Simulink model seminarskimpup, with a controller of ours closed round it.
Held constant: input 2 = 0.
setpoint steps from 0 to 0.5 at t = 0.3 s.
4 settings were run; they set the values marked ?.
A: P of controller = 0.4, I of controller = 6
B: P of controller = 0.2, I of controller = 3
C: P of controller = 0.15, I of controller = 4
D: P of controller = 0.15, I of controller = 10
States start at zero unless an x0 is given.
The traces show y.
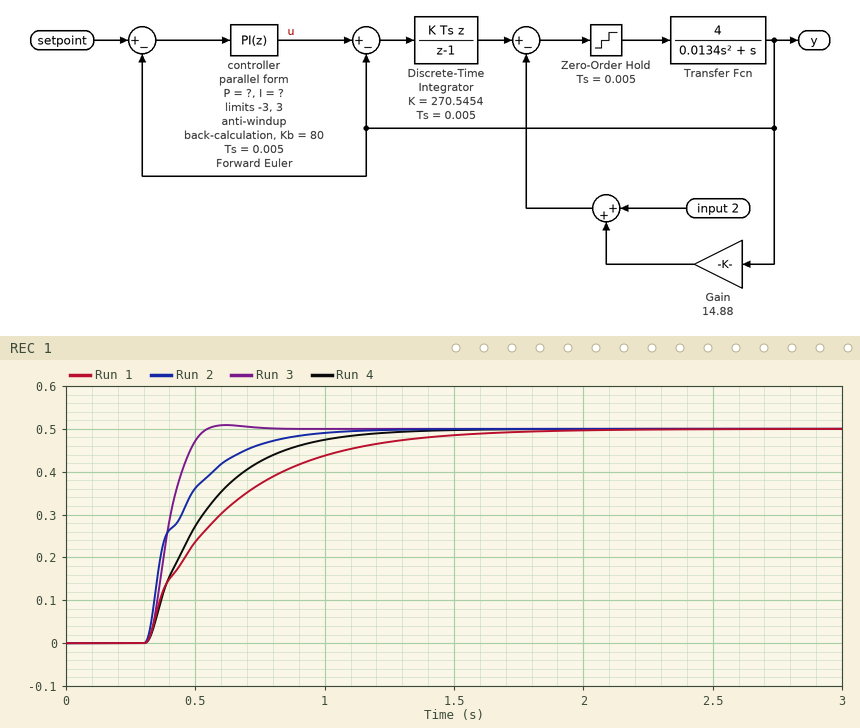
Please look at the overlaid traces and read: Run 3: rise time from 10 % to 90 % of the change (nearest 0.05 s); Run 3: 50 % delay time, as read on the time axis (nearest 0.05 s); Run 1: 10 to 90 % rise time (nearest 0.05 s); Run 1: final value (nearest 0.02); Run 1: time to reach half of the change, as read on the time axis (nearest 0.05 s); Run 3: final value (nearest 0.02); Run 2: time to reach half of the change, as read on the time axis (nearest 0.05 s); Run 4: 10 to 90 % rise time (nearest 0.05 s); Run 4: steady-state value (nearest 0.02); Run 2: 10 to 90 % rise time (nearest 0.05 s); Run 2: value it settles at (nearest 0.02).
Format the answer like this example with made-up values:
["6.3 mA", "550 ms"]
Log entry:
["0.15 s", "0.40 s", "0.75 s", "0.50", "0.50 s", "0.50", "0.40 s", "0.50 s", "0.50", "0.35 s", "0.50"]
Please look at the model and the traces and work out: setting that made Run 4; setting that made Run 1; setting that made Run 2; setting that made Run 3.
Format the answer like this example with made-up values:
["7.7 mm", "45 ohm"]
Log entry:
["C", "B", "A", "D"]
